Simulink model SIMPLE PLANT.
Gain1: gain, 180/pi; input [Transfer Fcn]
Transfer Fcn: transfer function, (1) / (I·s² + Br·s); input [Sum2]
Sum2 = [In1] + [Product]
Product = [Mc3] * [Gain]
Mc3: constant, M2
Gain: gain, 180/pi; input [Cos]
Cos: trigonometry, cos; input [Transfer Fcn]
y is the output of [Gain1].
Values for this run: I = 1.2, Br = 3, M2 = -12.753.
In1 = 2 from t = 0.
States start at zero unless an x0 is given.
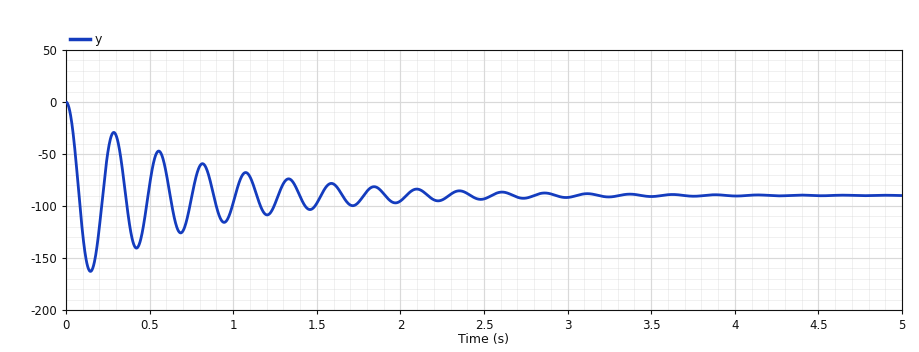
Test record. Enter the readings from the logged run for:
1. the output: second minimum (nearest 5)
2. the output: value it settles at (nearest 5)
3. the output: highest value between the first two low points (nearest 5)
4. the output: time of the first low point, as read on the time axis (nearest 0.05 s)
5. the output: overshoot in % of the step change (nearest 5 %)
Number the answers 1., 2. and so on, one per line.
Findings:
1. -140
2. -90
3. -30
4. 0.15 s
5. 80 %
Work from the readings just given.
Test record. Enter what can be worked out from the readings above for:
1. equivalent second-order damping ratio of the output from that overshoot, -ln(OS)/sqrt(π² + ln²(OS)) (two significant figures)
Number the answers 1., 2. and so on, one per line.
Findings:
1. 0.071
